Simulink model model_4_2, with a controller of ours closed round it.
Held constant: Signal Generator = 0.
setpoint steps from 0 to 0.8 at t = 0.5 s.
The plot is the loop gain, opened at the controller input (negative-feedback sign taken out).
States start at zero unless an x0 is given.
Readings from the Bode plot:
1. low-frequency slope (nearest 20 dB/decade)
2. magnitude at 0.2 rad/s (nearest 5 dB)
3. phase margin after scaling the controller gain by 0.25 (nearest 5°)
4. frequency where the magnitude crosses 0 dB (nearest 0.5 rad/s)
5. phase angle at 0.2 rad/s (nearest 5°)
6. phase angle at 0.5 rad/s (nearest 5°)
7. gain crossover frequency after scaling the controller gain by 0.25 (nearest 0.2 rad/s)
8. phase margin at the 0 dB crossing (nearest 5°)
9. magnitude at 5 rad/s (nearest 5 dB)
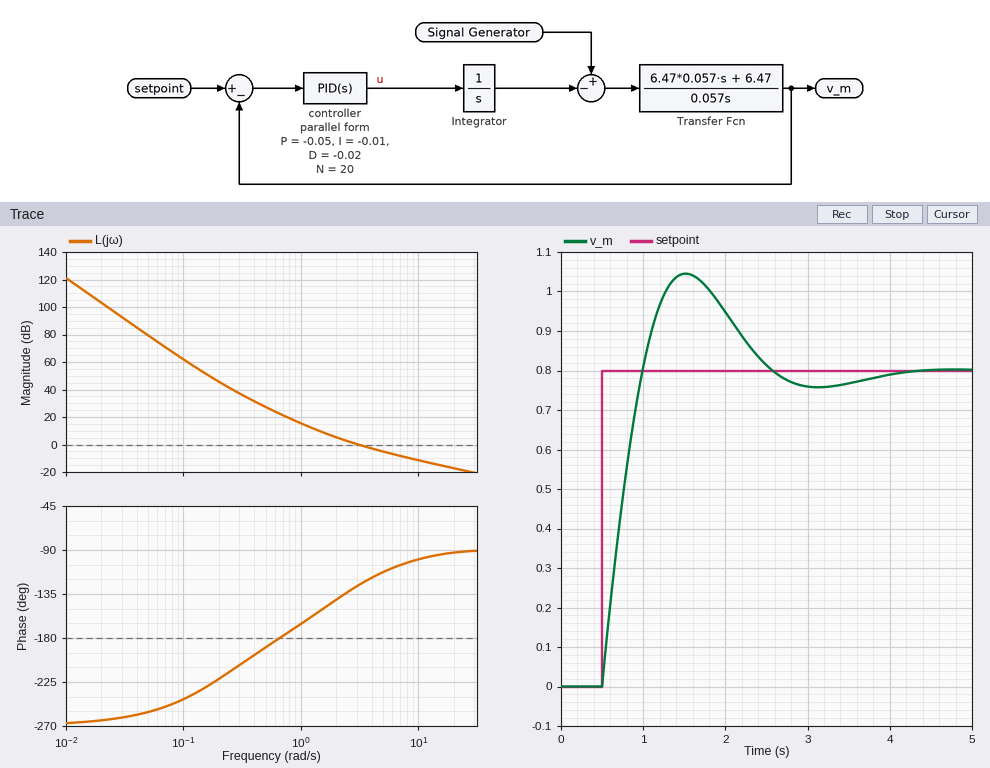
-60 dB/decade
45 dB
20°
3.0 rad/s
-220°
-190°
1.2 rad/s
55°
-5 dB
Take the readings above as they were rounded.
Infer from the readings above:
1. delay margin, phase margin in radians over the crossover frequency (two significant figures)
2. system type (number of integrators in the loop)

0.32 s
3
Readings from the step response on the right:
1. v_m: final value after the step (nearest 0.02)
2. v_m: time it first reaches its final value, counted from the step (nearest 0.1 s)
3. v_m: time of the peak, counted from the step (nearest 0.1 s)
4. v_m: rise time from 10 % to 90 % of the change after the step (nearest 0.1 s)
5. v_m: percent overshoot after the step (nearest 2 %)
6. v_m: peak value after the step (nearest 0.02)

0.80
0.5 s
1.0 s
0.4 s
30 %
1.04
